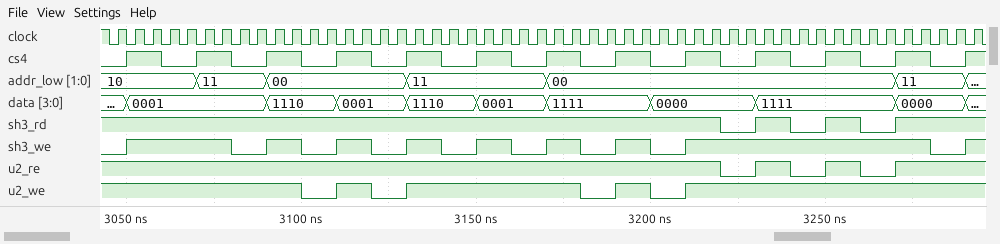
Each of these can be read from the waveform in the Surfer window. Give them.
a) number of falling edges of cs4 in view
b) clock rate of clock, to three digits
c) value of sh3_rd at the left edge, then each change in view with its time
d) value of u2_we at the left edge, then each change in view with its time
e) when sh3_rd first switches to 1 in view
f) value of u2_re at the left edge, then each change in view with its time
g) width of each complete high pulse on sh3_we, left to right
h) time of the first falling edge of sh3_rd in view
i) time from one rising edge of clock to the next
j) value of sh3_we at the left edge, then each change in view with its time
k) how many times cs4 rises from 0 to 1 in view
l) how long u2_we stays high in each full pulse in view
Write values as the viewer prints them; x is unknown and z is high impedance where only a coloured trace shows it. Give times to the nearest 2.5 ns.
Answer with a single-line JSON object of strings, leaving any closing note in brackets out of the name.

{"number of falling edges of cs4 in view": "12", "clock rate of clock, to three digits": "200 MHz", "value of sh3_rd at the left edge, then each change in view with its time": "1, 0 at 3220 ns, 1 at 3230 ns, 0 at 3240 ns, 1 at 3250 ns, 0 at 3260 ns, 1 at 3270 ns", "value of u2_we at the left edge, then each change in view with its time": "1, 0 at 3100 ns, 1 at 3110 ns, 0 at 3120 ns, 1 at 3130 ns, 0 at 3180 ns, 1 at 3190 ns, 0 at 3200 ns, 1 at 3210 ns", "when sh3_rd first switches to 1 in view": "3230 ns", "value of u2_re at the left edge, then each change in view with its time": "1, 0 at 3220 ns, 1 at 3230 ns, 0 at 3240 ns, 1 at 3250 ns, 0 at 3260 ns, 1 at 3270 ns", "width of each complete high pulse on sh3_we, left to right": "30 ns, 10 ns, 10 ns, 10 ns, 10 ns, 10 ns, 10 ns, 70 ns", "time of the first falling edge of sh3_rd in view": "3220 ns", "time from one rising edge of clock to the next": "5 ns", "value of sh3_we at the left edge, then each change in view with its time": "0, 1 at 3050 ns, 0 at 3080 ns, 1 at 3090 ns, 0 at 3100 ns, 1 at 3110 ns, 0 at 3120 ns, 1 at 3130 ns, 0 at 3140 ns, 1 at 3150 ns, 0 at 3160 ns, 1 at 3170 ns, 0 at 3180 ns, 1 at 3190 ns, 0 at 3200 ns, 1 at 3210 ns, 0 at 3280 ns, 1 at 3290 ns", "how many times cs4 rises from 0 to 1 in view": "13", "how long u2_we stays high in each full pulse in view": "10 ns, 50 ns, 10 ns"}
